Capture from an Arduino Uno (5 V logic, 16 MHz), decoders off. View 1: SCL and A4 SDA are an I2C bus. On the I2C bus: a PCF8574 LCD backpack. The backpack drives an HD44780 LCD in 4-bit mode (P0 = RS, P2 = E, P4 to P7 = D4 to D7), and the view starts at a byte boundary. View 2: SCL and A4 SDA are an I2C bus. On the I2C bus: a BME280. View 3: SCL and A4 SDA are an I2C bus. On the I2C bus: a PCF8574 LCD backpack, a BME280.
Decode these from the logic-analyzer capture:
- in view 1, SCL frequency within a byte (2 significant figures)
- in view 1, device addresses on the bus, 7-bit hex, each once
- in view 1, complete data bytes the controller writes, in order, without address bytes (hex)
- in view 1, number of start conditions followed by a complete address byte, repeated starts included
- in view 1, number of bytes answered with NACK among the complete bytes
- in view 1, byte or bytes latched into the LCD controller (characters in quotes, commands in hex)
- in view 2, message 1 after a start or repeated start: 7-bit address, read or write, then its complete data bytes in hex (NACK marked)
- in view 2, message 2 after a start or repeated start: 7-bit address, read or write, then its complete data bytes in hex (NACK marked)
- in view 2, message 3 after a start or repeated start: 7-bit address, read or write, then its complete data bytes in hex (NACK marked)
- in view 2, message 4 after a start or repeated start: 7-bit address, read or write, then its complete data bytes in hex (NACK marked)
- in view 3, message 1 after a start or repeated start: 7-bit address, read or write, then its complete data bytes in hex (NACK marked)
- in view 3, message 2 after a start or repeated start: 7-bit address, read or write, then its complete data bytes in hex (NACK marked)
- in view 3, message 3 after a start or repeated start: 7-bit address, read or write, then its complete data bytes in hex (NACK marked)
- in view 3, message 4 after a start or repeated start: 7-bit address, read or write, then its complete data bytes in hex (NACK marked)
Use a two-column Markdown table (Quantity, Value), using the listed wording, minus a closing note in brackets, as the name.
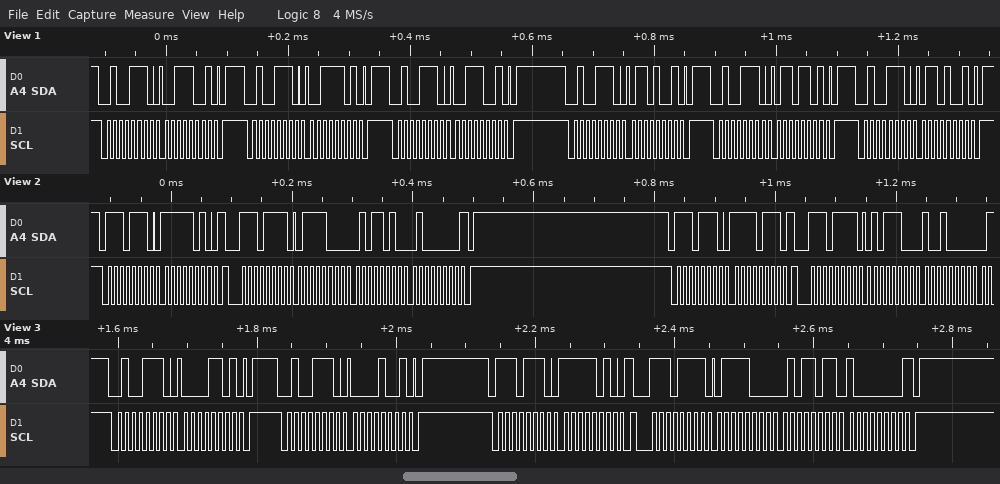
| Quantity | Value |
|---|---|
| in view 1, SCL frequency within a byte | 100 kHz |
| in view 1, device addresses on the bus, 7-bit hex, each once | 0x27 |
| in view 1, complete data bytes the controller writes, in order, without address bytes | 39 3D 39 69 6D 69 |
| in view 1, number of start conditions followed by a complete address byte, repeated starts included | 6 |
| in view 1, number of bytes answered with NACK among the complete bytes | 0 |
| in view 1, byte or bytes latched into the LCD controller | '6' |
| in view 2, message 1 after a start or repeated start: 7-bit address, read or write, then its complete data bytes in hex | 0x77 write: FA |
| in view 2, message 2 after a start or repeated start: 7-bit address, read or write, then its complete data bytes in hex | 0x77 read: 78 5A 40 NACK |
| in view 2, message 3 after a start or repeated start: 7-bit address, read or write, then its complete data bytes in hex | 0x77 write: F7 |
| in view 2, message 4 after a start or repeated start: 7-bit address, read or write, then its complete data bytes in hex | 0x77 read: 5C 90 |
| in view 3, message 1 after a start or repeated start: 7-bit address, read or write, then its complete data bytes in hex | 0x27 write: 0D |
| in view 3, message 2 after a start or repeated start: 7-bit address, read or write, then its complete data bytes in hex | 0x27 write: 09 |
| in view 3, message 3 after a start or repeated start: 7-bit address, read or write, then its complete data bytes in hex | 0x77 write: FA |
| in view 3, message 4 after a start or repeated start: 7-bit address, read or write, then its complete data bytes in hex | 0x77 read: 78 5B 80 NACK |
